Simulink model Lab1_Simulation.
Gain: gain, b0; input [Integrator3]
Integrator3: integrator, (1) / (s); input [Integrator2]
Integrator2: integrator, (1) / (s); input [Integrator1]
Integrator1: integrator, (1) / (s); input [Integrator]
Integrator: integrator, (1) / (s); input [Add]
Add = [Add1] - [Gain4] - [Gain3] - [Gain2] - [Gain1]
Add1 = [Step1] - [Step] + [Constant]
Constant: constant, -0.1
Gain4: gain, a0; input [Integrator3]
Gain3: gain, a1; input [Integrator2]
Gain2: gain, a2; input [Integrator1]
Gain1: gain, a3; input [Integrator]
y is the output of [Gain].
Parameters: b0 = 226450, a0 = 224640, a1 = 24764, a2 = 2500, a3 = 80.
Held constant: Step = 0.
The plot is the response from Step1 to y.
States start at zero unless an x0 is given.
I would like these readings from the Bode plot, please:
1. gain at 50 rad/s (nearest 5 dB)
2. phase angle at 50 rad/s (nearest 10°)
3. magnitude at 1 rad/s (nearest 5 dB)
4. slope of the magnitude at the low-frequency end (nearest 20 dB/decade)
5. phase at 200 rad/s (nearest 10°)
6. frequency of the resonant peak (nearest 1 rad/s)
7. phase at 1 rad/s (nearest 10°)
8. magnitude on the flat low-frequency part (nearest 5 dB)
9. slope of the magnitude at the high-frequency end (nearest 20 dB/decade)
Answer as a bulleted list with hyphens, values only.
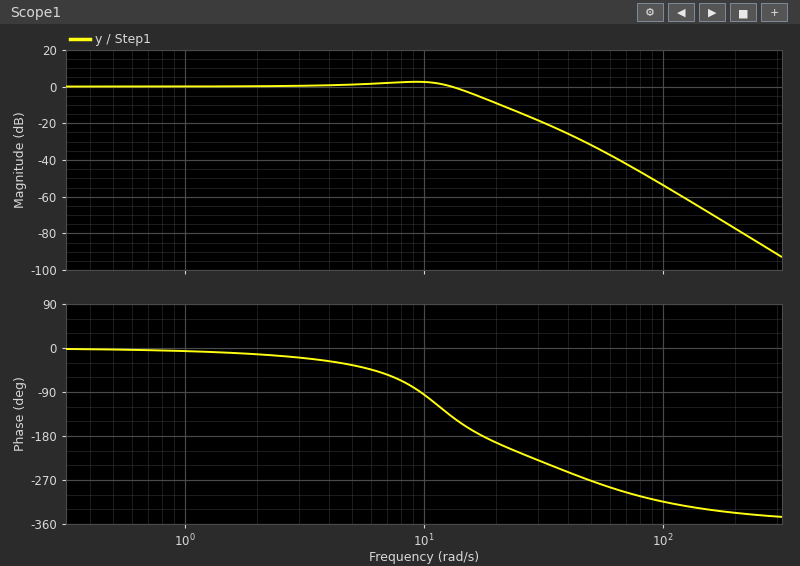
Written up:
- -30 dB
- -270°
- 0 dB
- 0 dB/decade
- -340°
- 9 rad/s
- -10°
- 0 dB
- -80 dB/decade
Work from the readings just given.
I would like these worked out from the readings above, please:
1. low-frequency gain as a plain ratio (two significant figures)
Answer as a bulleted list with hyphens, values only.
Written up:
- 1.0
